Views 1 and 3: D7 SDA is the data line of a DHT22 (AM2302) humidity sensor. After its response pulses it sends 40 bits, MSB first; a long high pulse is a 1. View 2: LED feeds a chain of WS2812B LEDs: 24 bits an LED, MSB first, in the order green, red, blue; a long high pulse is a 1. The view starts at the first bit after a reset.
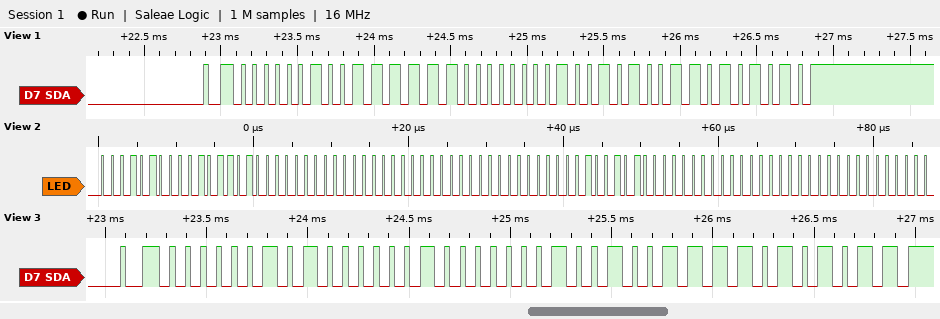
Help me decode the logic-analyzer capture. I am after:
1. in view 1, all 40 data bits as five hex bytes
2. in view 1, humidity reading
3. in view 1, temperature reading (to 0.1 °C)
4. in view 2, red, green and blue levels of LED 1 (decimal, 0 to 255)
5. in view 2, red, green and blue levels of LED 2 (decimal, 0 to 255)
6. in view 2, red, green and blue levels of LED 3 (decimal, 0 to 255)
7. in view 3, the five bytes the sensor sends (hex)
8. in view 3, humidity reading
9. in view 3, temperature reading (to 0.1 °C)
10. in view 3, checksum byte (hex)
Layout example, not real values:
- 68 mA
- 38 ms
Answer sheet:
- 02 7E 01 29 AA
- 63.8 %
- 29.7 °C
- 45, 20, 0
- 0, 0, 0
- 0, 37, 0
- 02 81 01 27 AB
- 64.1 %
- 29.5 °C
- 0xAB
